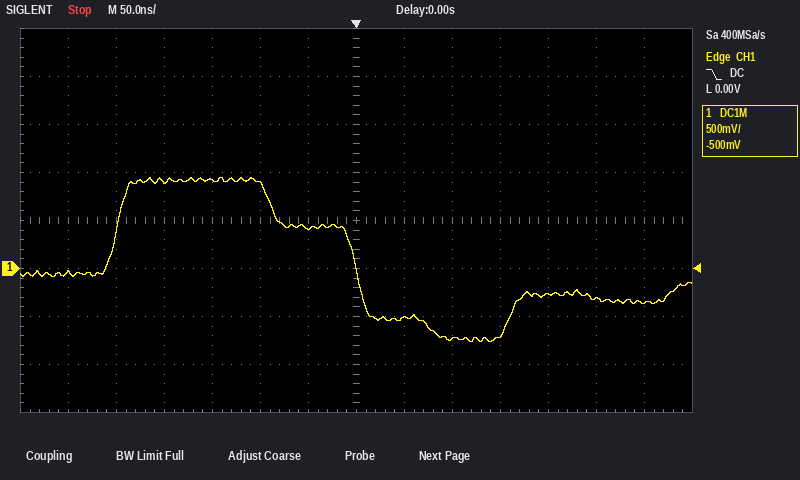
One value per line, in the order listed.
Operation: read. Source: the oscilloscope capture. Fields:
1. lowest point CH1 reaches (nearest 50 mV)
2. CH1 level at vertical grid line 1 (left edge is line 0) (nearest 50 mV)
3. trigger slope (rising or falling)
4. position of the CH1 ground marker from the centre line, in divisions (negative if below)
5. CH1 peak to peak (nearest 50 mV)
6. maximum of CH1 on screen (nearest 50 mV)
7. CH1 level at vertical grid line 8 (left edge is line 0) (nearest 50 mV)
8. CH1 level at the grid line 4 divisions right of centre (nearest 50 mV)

-750 mV
-50 mV
falling
-1.0 div
1.70 V
950 mV
-500 mV
-250 mV
